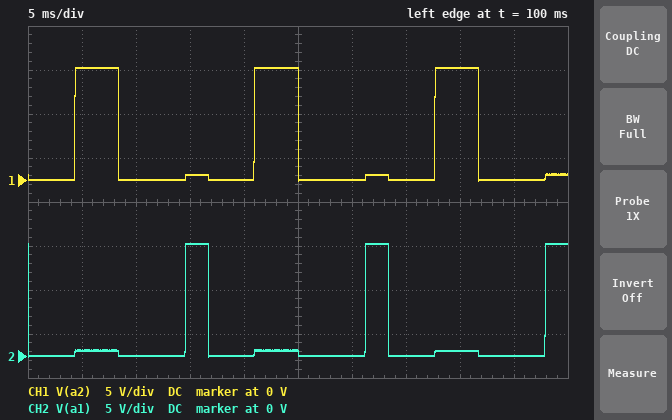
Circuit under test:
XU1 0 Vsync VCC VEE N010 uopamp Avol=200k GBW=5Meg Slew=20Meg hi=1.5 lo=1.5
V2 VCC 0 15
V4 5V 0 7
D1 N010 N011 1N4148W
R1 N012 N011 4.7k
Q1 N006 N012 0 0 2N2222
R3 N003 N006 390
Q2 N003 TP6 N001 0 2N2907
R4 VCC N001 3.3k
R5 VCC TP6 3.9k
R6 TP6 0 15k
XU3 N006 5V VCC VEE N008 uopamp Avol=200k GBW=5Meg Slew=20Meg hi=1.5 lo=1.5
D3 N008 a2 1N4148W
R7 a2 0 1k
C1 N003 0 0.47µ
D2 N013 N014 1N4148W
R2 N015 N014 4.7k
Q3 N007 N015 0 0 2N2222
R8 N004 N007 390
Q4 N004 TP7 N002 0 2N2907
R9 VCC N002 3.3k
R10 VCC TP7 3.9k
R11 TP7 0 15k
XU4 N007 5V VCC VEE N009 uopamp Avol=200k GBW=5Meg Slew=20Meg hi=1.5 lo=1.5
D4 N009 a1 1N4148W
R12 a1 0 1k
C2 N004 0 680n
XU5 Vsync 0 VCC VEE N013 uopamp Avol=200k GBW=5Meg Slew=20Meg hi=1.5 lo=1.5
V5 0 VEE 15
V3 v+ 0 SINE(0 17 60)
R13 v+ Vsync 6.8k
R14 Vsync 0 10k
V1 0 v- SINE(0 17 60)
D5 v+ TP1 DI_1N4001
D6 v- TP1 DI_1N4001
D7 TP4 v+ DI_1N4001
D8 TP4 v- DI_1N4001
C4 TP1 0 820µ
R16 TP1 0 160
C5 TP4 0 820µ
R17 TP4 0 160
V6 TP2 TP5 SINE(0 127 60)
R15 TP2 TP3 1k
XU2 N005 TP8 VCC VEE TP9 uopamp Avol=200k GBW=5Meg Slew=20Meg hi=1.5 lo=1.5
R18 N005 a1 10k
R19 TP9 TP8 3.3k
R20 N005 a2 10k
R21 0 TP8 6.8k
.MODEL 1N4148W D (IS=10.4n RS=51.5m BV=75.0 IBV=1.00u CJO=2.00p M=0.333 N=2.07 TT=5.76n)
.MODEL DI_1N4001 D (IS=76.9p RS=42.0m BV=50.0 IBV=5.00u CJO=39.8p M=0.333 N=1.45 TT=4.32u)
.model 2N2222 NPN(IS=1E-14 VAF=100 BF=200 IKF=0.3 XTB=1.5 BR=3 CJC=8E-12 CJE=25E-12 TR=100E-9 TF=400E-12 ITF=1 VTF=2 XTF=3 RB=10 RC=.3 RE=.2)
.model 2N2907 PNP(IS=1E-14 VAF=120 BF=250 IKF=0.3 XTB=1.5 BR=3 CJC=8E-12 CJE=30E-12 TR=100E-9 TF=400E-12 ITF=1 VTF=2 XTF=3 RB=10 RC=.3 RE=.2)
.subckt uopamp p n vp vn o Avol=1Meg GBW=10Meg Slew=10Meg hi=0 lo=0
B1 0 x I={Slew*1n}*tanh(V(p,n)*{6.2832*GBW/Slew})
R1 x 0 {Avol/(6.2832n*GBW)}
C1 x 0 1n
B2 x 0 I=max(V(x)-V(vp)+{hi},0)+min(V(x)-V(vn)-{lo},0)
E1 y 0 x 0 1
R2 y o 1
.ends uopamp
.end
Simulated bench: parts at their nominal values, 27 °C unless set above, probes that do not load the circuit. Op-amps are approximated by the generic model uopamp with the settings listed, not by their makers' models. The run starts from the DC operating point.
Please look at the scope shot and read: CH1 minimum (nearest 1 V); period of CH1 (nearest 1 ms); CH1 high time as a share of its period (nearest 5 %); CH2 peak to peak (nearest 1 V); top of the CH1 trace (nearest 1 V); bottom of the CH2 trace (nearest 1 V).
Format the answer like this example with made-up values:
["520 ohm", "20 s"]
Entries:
["0 V", "17 ms", "25 %", "13 V", "13 V", "0 V"]
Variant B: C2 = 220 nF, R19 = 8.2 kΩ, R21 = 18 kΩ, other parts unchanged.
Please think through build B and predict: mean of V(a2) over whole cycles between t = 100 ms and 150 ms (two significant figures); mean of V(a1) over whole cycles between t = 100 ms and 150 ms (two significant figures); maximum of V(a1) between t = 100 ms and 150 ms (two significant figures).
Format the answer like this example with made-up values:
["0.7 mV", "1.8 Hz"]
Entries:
["3.3 V", "5.0 V", "13 V"]
